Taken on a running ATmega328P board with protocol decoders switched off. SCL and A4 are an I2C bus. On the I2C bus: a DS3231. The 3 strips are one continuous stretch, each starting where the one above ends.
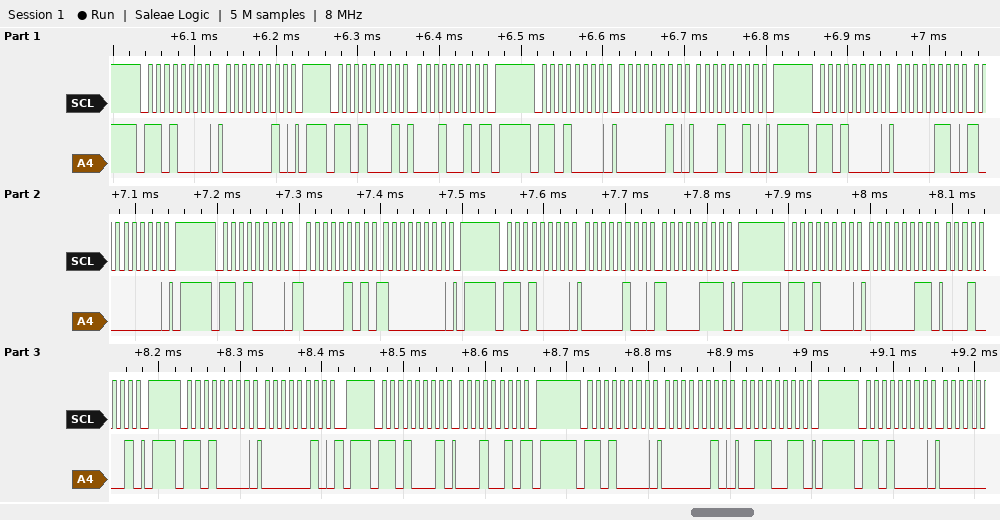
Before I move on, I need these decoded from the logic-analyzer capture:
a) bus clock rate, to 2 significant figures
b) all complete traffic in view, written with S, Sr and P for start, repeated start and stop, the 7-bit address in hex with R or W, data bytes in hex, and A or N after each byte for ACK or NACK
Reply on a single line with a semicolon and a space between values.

100 kHz; S 68W A 02 A P S 68R A 12 N P S 68W A 02 A 12 A P S 68W A 06 A 80 A P S 68W A 05 A 80 A P S 68W A 04 A 87 A P S 68W A 03 A 11 A P S 68W A 02 A P S 68R A 12 N P S 68W A 02 A 33 A P S 68W A
